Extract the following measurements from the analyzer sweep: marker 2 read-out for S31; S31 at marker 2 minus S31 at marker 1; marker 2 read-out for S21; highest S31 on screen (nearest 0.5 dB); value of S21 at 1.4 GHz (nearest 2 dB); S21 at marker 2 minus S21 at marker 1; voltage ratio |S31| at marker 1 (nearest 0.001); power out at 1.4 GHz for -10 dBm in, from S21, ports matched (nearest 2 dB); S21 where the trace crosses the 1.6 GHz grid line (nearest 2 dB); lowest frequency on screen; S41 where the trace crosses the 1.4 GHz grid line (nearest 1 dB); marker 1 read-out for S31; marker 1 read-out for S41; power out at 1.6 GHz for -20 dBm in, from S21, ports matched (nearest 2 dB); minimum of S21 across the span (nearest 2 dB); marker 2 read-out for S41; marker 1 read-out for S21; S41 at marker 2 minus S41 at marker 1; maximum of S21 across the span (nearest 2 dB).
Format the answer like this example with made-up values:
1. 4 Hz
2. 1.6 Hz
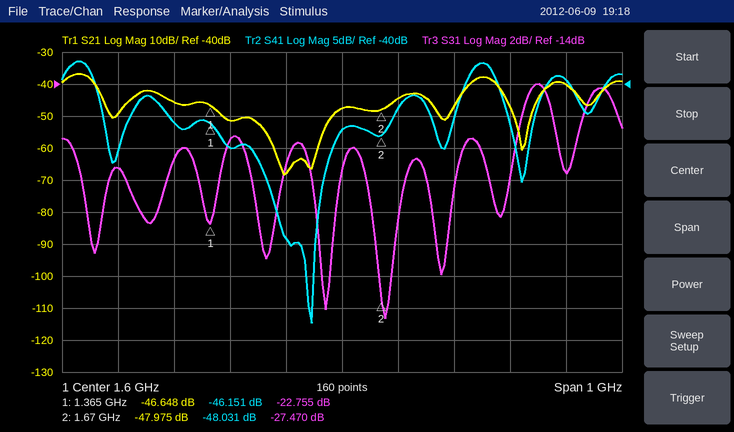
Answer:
1. -27.470 dB
2. -4.715 dB
3. -47.975 dB
4. -14.0 dB
5. -52 dB
6. -1.327 dB
7. 0.073
8. -62 dBm
9. -48 dB
10. 1.1 GHz
11. -50 dB
12. -22.755 dB
13. -46.151 dB
14. -68 dBm
15. -68 dB
16. -48.031 dB
17. -46.648 dB
18. -1.880 dB
19. -36 dB
